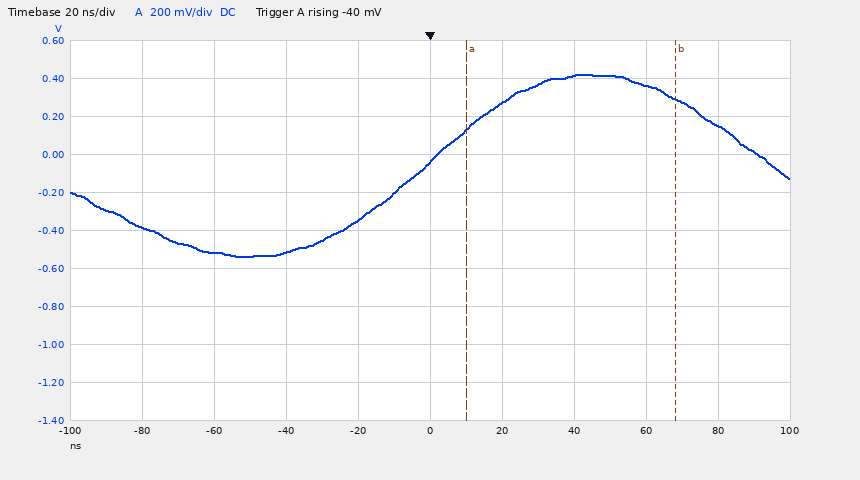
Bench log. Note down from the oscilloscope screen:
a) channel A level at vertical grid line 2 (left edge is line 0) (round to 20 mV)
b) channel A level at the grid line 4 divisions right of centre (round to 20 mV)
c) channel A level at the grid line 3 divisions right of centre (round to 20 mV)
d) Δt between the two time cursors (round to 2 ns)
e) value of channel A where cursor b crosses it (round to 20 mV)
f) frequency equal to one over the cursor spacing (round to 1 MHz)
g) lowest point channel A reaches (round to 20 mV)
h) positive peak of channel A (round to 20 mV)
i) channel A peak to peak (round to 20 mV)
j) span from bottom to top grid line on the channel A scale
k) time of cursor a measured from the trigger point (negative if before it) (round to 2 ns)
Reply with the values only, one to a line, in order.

-520 mV
160 mV
360 mV
58 ns
300 mV
17 MHz
-540 mV
420 mV
960 mV
2 V
+10 ns
